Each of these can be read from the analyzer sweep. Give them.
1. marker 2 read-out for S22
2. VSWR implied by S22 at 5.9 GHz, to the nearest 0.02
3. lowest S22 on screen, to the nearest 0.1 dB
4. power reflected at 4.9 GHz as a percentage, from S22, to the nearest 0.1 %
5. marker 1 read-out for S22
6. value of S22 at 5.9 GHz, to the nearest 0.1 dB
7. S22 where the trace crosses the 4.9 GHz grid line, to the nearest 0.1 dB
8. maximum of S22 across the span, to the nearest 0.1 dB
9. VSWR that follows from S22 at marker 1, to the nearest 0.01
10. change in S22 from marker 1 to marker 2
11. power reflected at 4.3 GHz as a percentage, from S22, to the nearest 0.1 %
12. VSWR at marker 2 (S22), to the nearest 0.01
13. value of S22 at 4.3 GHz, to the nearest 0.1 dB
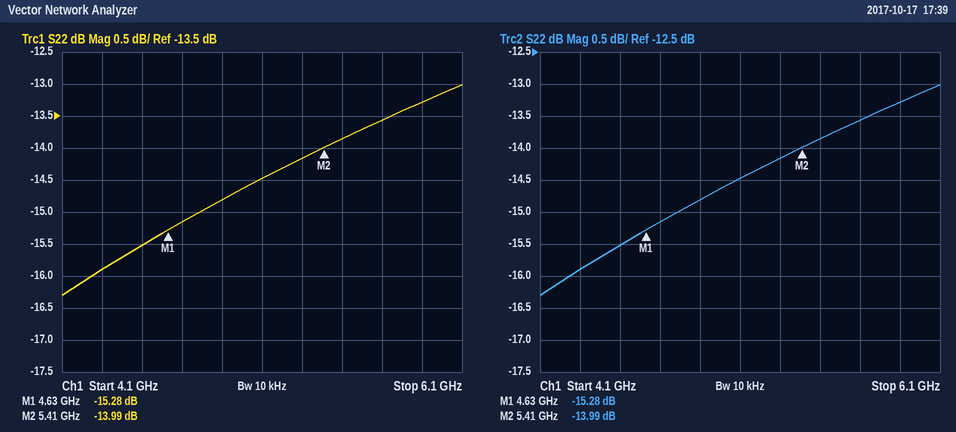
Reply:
-13.99 dB
1.56
-16.3 dB
3.3 %
-15.28 dB
-13.3 dB
-14.8 dB
-13.0 dB
1.42
1.29 dB
2.6 %
1.50
-15.9 dB
